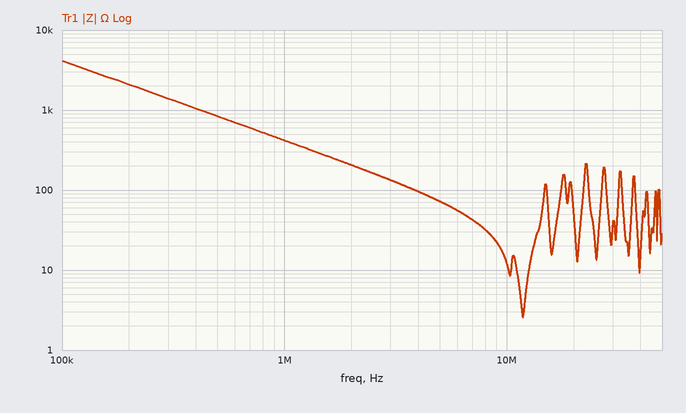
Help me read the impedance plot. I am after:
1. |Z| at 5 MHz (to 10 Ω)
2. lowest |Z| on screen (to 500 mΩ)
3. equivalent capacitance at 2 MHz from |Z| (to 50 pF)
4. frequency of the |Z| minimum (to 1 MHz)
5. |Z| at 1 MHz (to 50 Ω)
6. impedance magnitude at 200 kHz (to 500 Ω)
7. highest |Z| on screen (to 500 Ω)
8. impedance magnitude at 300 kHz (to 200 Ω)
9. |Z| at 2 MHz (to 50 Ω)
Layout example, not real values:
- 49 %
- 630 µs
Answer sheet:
- 70 Ω
- 2.5 Ω
- 400 pF
- 12 MHz
- 400 Ω
- 2.0 kΩ
- 4.0 kΩ
- 1.4 kΩ
- 200 Ω
